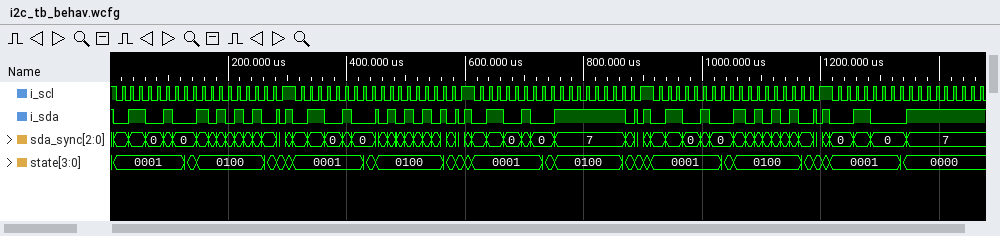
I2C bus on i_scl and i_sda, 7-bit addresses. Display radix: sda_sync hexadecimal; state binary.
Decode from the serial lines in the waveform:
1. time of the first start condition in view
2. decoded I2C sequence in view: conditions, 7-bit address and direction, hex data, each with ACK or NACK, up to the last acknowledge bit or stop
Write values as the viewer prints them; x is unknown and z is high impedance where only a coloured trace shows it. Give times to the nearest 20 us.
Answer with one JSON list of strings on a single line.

["0 us", "start, address 32 write ACK, AA ACK, stop, start, address 32 write ACK, 55 ACK, stop, start, address 32 write ACK, FF ACK, stop, start, address 32 write ACK, AA ACK, stop, start, address 18 write NACK"]
